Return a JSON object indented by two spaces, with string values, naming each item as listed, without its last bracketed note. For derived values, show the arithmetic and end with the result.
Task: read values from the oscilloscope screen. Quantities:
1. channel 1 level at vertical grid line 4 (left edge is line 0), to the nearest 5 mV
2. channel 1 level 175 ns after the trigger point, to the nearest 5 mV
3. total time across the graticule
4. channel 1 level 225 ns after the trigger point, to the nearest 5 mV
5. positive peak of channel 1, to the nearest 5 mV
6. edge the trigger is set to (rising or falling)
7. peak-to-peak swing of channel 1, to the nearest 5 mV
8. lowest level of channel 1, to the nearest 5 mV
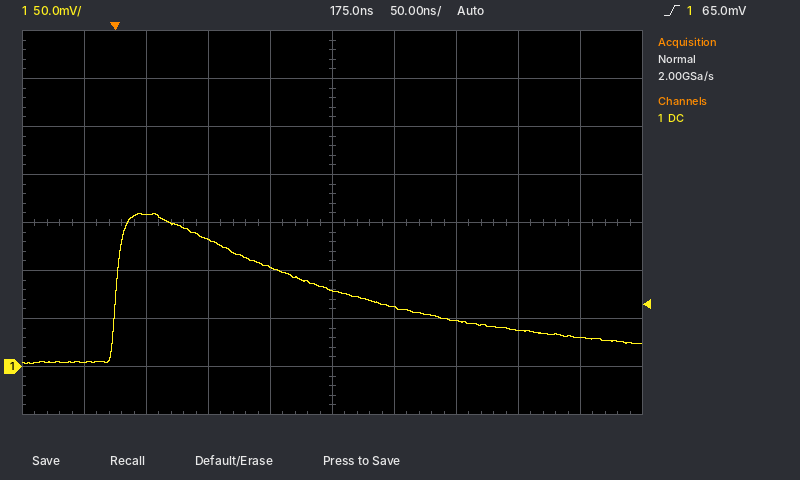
{
  "channel 1 level at vertical grid line 4 (left edge is line 0), to the nearest 5 mV": "105 mV",
  "channel 1 level 175 ns after the trigger point, to the nearest 5 mV": "80 mV",
  "total time across the graticule": "500 ns",
  "channel 1 level 225 ns after the trigger point, to the nearest 5 mV": "60 mV",
  "positive peak of channel 1, to the nearest 5 mV": "160 mV",
  "edge the trigger is set to": "rising",
  "peak-to-peak swing of channel 1, to the nearest 5 mV": "160 mV − (5 mV) = 155 mV",
  "lowest level of channel 1, to the nearest 5 mV": "5 mV"
}
